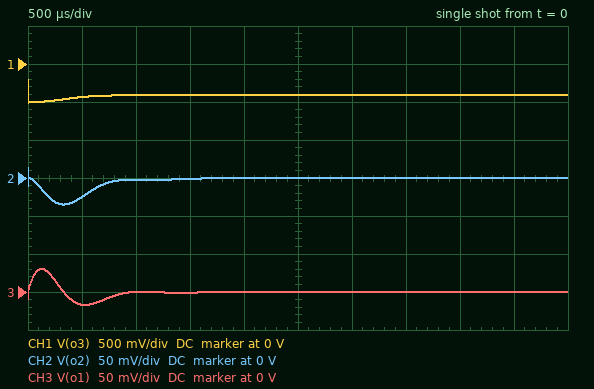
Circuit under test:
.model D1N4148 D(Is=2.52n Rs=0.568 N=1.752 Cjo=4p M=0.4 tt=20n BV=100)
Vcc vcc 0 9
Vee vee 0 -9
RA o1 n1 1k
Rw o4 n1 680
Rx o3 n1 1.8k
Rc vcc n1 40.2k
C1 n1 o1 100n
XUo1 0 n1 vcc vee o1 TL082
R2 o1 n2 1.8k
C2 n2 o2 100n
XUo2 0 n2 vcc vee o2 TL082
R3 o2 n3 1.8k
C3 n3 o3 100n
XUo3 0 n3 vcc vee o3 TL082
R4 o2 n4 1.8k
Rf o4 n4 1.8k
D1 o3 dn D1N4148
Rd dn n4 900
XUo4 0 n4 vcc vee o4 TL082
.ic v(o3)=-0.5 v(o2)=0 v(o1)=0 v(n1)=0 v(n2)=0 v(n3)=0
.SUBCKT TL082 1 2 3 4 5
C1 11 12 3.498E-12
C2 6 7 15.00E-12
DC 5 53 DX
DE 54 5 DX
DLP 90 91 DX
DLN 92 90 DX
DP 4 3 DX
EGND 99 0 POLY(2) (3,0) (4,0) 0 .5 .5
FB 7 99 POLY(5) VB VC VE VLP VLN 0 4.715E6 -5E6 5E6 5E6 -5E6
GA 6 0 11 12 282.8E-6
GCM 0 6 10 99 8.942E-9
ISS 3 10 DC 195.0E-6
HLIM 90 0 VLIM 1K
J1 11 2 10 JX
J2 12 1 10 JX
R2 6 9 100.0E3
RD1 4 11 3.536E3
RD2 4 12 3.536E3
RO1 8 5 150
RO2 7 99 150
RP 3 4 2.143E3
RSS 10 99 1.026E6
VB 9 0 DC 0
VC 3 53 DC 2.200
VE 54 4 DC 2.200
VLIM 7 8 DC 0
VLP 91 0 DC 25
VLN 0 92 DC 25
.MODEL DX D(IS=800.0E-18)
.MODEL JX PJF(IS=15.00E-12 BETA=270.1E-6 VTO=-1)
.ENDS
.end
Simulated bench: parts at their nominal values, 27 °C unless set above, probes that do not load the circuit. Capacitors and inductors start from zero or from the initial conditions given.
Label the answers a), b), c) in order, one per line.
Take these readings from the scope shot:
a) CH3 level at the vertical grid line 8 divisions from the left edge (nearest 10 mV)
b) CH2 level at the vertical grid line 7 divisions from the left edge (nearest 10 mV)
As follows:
a) 0 V
b) 0 V
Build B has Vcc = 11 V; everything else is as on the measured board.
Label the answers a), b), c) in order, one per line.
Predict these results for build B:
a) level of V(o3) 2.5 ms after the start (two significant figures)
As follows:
a) -490 mV
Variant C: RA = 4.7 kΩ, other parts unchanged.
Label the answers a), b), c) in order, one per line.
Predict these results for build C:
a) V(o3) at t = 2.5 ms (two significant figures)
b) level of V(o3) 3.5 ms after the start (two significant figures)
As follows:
a) -390 mV
b) -410 mV
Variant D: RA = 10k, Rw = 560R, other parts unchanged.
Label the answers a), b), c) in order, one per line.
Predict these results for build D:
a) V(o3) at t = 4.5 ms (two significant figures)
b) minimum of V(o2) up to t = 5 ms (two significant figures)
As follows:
a) -480 mV
b) -160 mV
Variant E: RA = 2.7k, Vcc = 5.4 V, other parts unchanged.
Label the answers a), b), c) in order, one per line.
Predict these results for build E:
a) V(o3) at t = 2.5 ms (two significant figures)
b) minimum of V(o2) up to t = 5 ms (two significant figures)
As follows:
a) -240 mV
b) -130 mV
